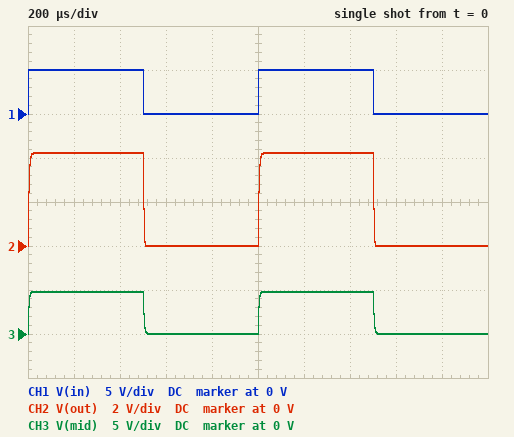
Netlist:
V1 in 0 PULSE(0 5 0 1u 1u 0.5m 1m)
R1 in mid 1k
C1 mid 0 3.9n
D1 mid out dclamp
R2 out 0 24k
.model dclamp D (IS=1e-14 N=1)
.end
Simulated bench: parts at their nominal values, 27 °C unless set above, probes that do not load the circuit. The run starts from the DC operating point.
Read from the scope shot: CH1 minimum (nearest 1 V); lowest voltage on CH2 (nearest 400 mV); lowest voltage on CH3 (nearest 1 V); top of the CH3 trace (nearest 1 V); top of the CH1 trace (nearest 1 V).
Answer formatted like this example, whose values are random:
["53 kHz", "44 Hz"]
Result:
["0 V", "0 V", "0 V", "5 V", "5 V"]
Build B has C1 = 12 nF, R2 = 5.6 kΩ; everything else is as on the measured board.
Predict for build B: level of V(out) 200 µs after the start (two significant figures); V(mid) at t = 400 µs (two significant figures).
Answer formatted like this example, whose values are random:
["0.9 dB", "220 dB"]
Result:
["3.7 V", "4.3 V"]
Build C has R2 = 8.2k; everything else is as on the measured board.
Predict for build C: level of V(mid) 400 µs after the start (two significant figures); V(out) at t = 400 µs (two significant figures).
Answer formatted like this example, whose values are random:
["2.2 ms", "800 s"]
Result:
["4.5 V", "3.9 V"]
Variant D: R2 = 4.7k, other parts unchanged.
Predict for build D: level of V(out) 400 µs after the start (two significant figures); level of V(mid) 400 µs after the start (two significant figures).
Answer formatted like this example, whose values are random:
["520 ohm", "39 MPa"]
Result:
["3.6 V", "4.2 V"]
